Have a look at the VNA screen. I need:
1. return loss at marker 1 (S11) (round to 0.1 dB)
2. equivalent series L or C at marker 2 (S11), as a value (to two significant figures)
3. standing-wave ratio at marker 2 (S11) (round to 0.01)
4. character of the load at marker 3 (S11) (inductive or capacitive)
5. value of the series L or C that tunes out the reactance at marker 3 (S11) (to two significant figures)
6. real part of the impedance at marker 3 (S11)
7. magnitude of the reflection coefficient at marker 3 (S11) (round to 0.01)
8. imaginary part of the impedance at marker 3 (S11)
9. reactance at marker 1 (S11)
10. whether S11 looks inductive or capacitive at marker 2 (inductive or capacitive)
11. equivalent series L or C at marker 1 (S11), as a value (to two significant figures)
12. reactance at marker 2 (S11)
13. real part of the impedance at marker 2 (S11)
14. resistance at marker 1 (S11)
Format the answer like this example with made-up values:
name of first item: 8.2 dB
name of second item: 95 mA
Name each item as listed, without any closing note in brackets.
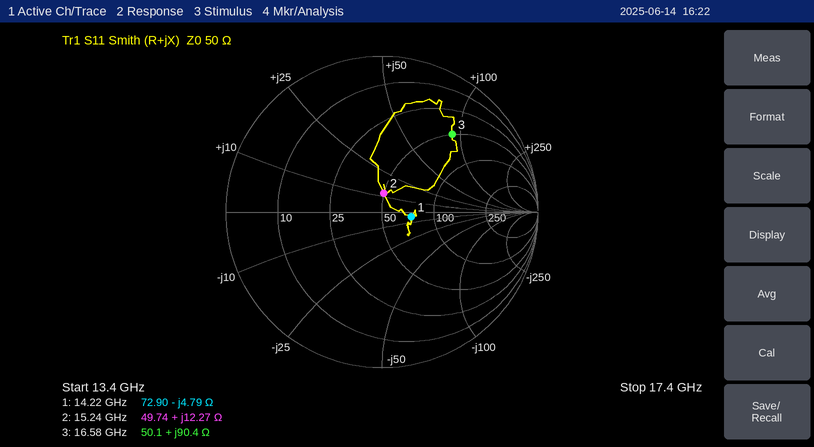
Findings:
return loss at marker 1 (S11): 14.4 dB
equivalent series L or C at marker 2 (S11), as a value: 130 pH
standing-wave ratio at marker 2 (S11): 1.28
character of the load at marker 3 (S11): inductive
value of the series L or C that tunes out the reactance at marker 3 (S11): 110 fF
real part of the impedance at marker 3: 50.1 Ω
magnitude of the reflection coefficient at marker 3 (S11): 0.67
imaginary part of the impedance at marker 3: +90.4 Ω
reactance at marker 1: -4.79 Ω
whether S11 looks inductive or capacitive at marker 2: inductive
equivalent series L or C at marker 1 (S11), as a value: 2.3 pF
reactance at marker 2: +12.27 Ω
real part of the impedance at marker 2: 49.74 Ω
resistance at marker 1: 72.90 Ω
